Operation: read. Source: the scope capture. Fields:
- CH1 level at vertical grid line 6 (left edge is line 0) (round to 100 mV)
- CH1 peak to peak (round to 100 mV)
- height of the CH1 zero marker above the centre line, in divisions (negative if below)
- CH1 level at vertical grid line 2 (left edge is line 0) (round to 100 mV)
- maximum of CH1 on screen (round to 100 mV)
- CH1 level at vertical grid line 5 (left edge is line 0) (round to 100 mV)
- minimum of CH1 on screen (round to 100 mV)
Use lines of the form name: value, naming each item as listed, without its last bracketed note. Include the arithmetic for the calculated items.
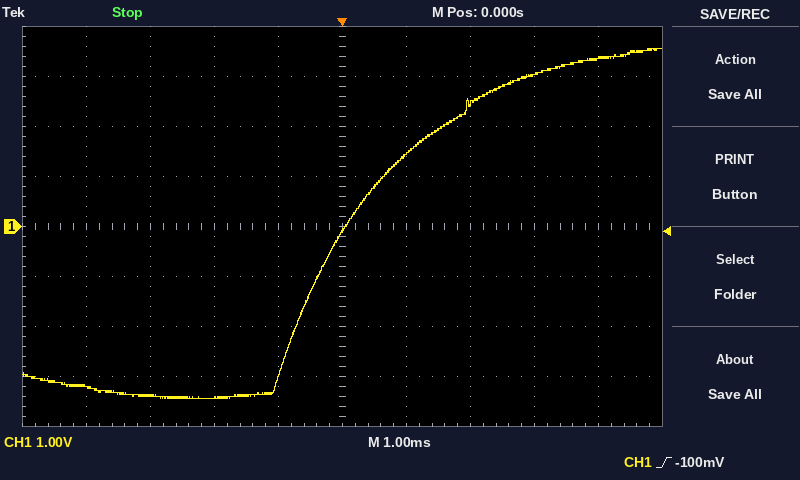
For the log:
CH1 level at vertical grid line 6 (left edge is line 0): 1.4 V
CH1 peak to peak: 3.6 V − (-3.4 V) = 7.0 V
height of the CH1 zero marker above the centre line, in divisions: 0.0 div
CH1 level at vertical grid line 2 (left edge is line 0): -3.4 V
maximum of CH1 on screen: 3.6 V
CH1 level at vertical grid line 5 (left edge is line 0): -100 mV
minimum of CH1 on screen: -3.4 V
